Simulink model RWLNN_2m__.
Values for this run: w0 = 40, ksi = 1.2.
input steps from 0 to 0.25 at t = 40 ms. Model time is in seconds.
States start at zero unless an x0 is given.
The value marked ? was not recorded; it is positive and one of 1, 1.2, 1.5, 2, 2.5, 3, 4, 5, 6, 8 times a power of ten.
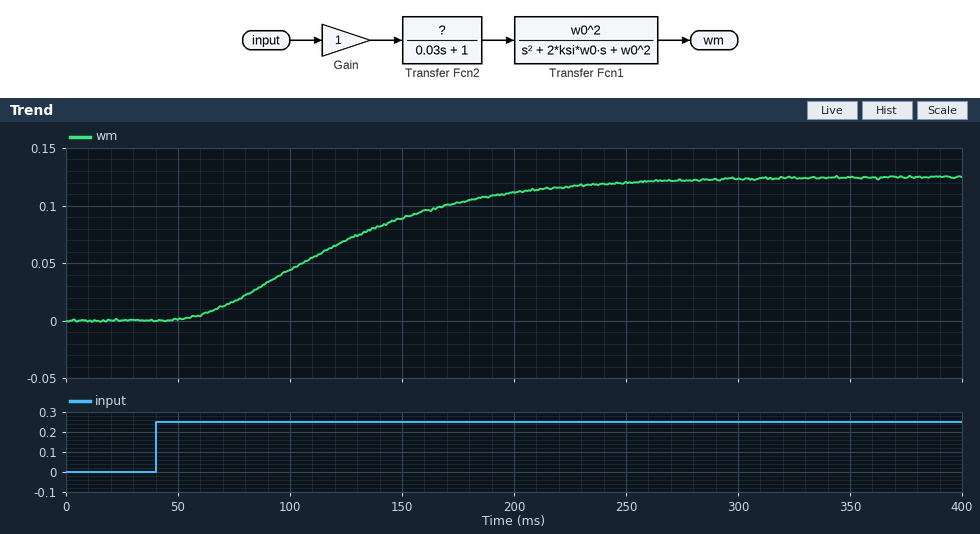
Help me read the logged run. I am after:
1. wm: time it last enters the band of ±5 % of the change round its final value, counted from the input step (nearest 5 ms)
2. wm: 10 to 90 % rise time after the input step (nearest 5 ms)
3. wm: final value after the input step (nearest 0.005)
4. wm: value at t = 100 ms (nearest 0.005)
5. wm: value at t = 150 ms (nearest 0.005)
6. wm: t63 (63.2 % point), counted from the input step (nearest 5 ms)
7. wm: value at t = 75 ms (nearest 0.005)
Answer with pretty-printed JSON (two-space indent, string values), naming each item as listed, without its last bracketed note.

{
  "wm: time it last enters the band of ±5 % of the change round its final value, counted from the input step": "200 ms",
  "wm: 10 to 90 % rise time after the input step": "135 ms",
  "wm: final value after the input step": "0.125",
  "wm: value at t = 100 ms": "0.045",
  "wm: value at t = 150 ms": "0.090",
  "wm: t63 (63.2 % point), counted from the input step": "95 ms",
  "wm: value at t = 75 ms": "0.015"
}
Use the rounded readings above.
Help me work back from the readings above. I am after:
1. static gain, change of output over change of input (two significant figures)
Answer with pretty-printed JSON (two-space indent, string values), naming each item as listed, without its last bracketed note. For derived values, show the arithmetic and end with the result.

{
  "static gain, change of output over change of input": "(0.125 - 0) / (0.25 - 0) = 0.50"
}
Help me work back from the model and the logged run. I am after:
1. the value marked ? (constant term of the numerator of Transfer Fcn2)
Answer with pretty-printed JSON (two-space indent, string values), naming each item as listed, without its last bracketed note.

{
  "the value marked ?": "0.5"
}
